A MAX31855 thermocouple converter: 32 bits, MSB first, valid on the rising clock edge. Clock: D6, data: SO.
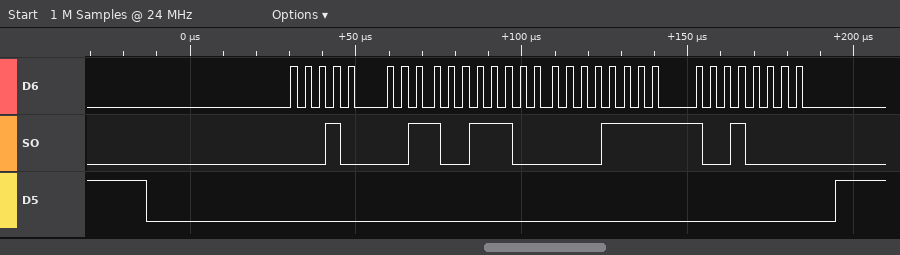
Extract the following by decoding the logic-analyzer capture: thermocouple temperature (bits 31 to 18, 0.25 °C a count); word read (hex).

281.75 °C
0x119C0F90
